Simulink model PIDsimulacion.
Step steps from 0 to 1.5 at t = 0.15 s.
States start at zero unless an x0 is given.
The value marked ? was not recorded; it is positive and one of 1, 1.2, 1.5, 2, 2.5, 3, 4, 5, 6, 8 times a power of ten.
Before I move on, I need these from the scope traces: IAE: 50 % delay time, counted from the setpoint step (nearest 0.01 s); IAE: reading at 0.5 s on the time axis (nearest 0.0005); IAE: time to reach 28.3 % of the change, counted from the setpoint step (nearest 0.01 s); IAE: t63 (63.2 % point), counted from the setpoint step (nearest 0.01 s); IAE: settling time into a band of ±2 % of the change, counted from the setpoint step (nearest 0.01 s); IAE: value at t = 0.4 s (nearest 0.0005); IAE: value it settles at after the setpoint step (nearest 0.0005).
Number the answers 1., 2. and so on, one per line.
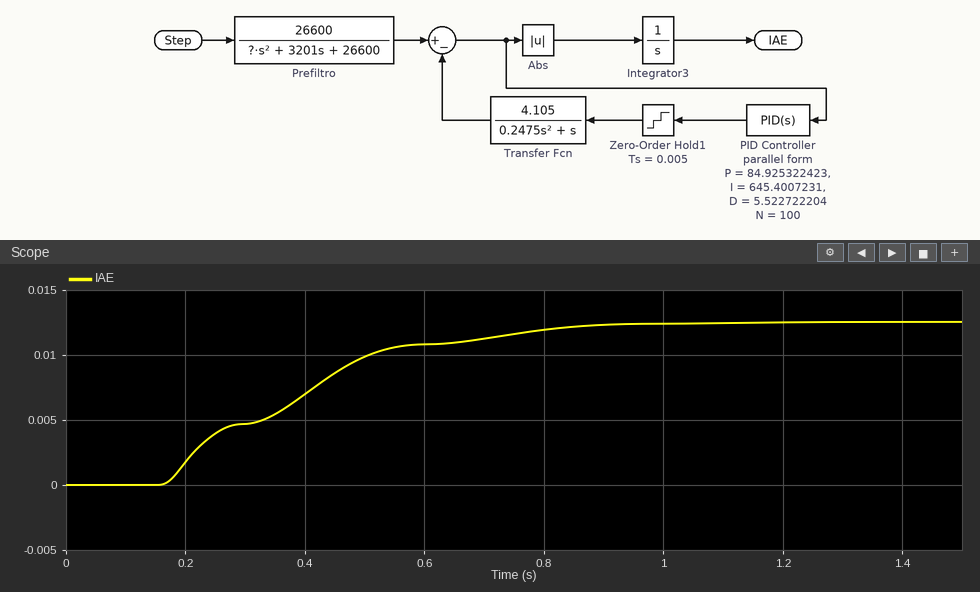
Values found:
1. 0.23 s
2. 0.0100
3. 0.09 s
4. 0.28 s
5. 0.74 s
6. 0.0070
7. 0.0125
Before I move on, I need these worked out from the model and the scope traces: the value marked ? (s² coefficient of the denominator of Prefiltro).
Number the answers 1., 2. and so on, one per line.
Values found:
1. 200
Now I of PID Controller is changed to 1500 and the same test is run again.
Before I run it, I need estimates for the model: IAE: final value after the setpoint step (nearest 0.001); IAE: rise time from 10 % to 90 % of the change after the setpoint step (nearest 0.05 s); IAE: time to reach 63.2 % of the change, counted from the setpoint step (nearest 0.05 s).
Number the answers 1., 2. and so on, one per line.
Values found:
1. 0.011
2. 0.40 s
3. 0.25 s
